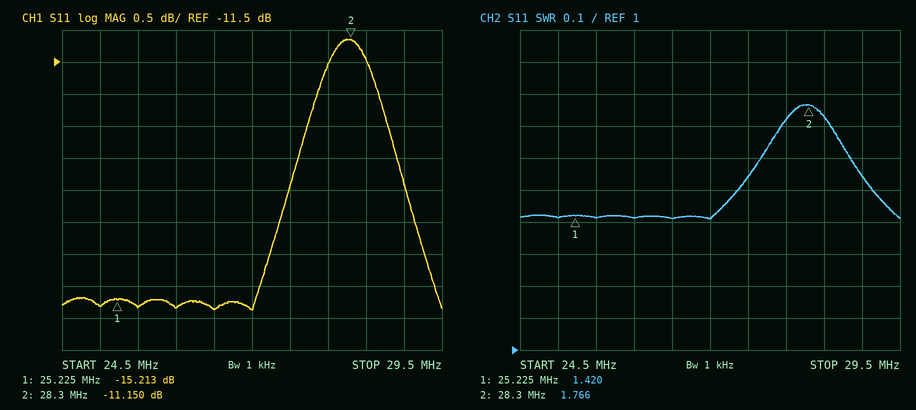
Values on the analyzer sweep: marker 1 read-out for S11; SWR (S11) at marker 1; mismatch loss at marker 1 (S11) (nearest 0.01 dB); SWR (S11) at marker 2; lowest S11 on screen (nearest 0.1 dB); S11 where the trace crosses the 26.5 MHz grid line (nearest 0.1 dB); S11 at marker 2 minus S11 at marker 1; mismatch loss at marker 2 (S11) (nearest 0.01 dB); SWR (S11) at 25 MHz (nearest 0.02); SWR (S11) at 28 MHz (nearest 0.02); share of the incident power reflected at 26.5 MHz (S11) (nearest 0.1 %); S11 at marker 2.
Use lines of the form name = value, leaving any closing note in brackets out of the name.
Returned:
marker 1 read-out for S11 = -15.213 dB
SWR (S11) at marker 1 = 1.420
mismatch loss at marker 1 (S11) = 0.13 dB
SWR (S11) at marker 2 = 1.766
lowest S11 on screen = -15.4 dB
S11 where the trace crosses the 26.5 MHz grid line = -15.4 dB
S11 at marker 2 minus S11 at marker 1 = 4.063 dB
mismatch loss at marker 2 (S11) = 0.35 dB
SWR (S11) at 25 MHz = 1.42
SWR (S11) at 28 MHz = 1.72
share of the incident power reflected at 26.5 MHz (S11) = 2.9 %
S11 at marker 2 = -11.150 dB
